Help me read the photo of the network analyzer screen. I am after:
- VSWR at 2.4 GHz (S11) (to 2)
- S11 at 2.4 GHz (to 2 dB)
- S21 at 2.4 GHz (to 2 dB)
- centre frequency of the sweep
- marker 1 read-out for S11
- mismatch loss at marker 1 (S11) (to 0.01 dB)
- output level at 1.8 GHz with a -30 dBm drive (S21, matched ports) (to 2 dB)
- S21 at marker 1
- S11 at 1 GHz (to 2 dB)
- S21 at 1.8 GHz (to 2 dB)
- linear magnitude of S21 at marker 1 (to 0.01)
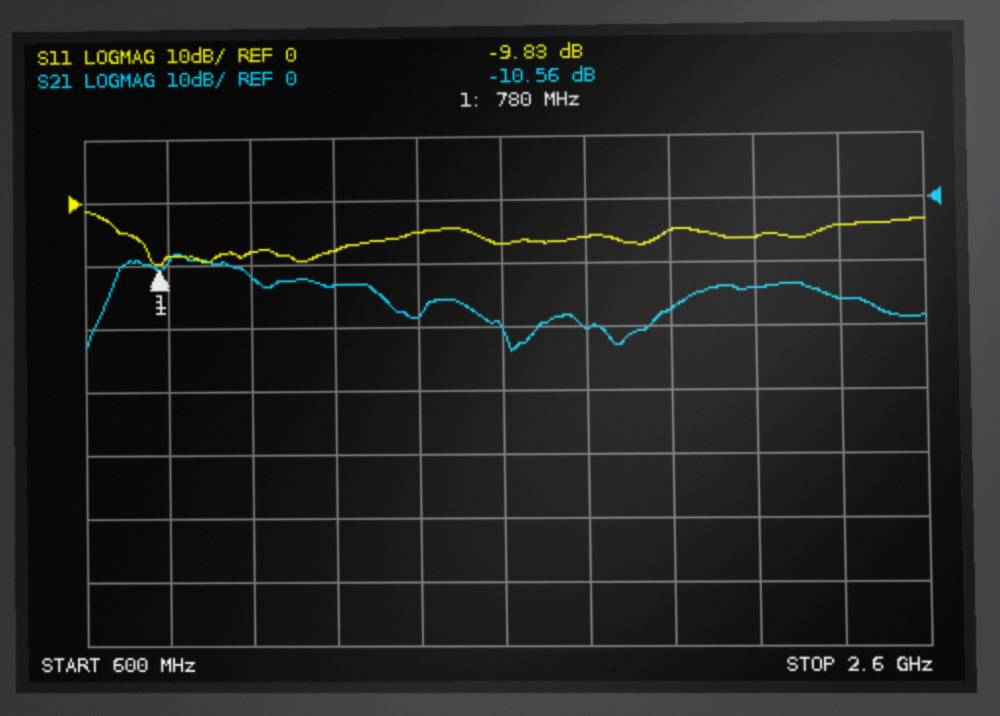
4
-4 dB
-16 dB
1.6 GHz
-9.83 dB
0.48 dB
-50 dBm
-10.56 dB
-8 dB
-20 dB
0.30
